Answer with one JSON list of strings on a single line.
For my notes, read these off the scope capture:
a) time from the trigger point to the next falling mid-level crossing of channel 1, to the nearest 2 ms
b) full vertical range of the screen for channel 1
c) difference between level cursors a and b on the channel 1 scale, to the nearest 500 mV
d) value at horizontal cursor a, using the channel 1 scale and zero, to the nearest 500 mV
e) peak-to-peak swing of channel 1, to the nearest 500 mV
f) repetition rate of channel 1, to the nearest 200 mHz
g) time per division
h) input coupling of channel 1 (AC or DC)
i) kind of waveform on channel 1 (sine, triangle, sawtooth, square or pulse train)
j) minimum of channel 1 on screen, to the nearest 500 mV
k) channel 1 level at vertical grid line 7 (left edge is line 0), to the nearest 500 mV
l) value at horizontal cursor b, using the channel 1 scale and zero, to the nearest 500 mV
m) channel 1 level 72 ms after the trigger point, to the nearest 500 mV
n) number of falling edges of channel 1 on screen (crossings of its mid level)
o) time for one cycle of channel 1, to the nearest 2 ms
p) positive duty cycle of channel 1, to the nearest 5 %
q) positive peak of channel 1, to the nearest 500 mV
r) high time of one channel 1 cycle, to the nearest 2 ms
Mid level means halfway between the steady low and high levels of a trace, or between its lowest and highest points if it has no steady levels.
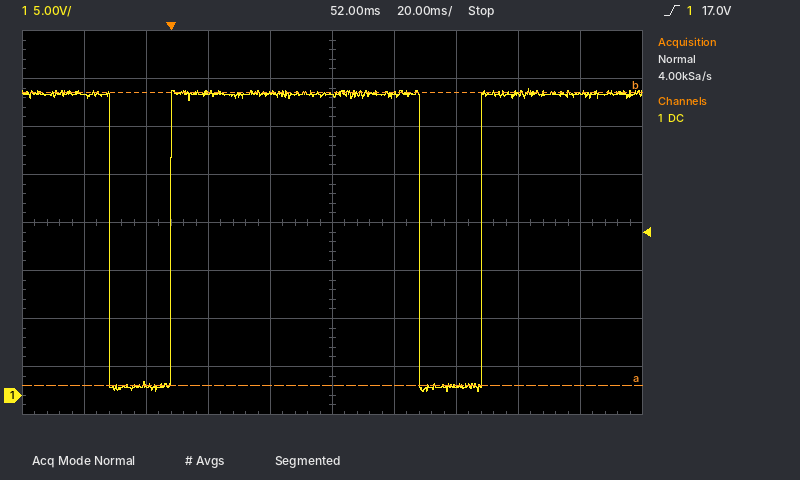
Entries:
["80 ms", "40 V", "30.5 V", "1.0 V", "31.5 V", "10.0 Hz", "20 ms", "DC", "pulse train", "500 mV", "1.0 V", "31.5 V", "31.5 V", "2", "100 ms", "80 %", "32.0 V", "80 ms"]
